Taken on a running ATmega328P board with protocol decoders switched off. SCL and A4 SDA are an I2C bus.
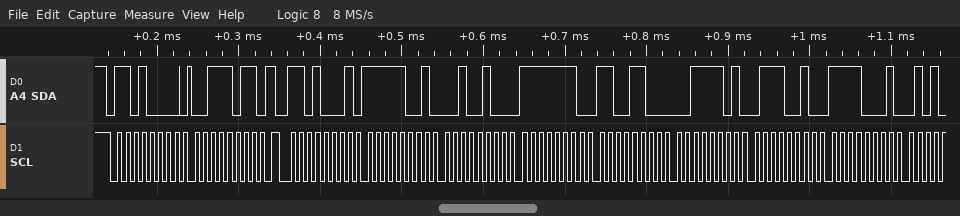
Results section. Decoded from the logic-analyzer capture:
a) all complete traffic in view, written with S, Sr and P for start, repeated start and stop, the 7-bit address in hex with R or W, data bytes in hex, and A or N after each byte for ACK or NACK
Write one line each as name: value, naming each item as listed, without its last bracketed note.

all complete traffic in view, written with S, Sr and P for start, repeated start and stop, the 7-bit address in hex with R or W, data bytes in hex, and A or N after each byte for ACK or NACK: S 68W A 3B A Sr 68R A F9 A 24 A FE A CC A 3D A 72 A F1 A
